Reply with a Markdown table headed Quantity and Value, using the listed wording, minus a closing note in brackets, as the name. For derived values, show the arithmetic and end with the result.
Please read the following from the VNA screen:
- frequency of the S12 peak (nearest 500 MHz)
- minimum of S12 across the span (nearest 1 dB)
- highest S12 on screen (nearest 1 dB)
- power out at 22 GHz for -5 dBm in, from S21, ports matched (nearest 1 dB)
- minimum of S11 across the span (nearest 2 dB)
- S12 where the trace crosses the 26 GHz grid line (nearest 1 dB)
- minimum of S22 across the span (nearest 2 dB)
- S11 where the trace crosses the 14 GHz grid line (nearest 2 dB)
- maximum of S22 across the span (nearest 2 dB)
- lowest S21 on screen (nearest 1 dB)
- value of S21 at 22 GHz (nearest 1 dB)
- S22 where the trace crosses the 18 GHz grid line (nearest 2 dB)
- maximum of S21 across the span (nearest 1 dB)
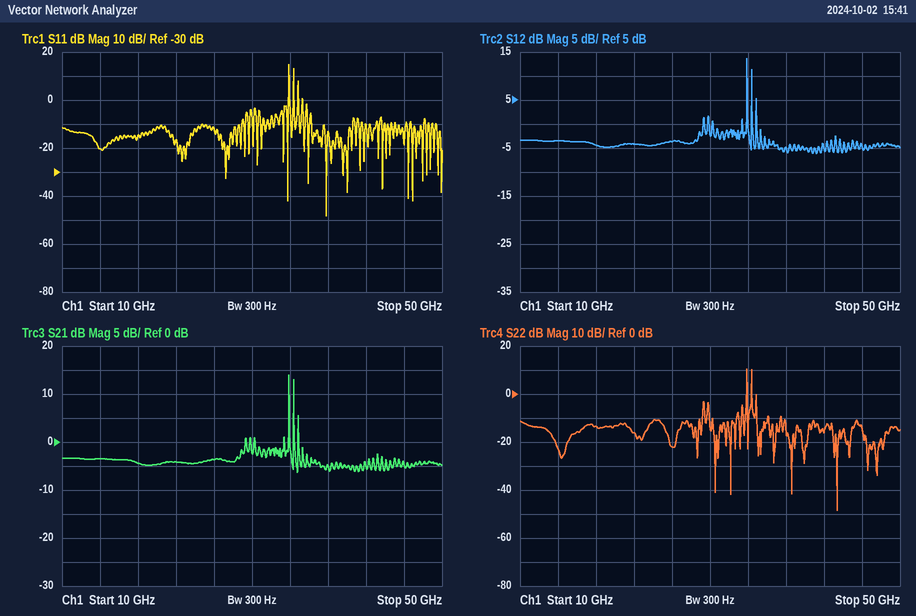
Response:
| Quantity | Value |
|---|---|
| frequency of the S12 peak | 34.0 GHz |
| minimum of S12 across the span | -6 dB |
| highest S12 on screen | 14 dB |
| power out at 22 GHz for -5 dBm in, from S21, ports matched | -5 dBm + (-4 dB) = -9 dBm |
| minimum of S11 across the span | -48 dB |
| S12 where the trace crosses the 26 GHz grid line | -4 dB |
| minimum of S22 across the span | -48 dB |
| S11 where the trace crosses the 14 GHz grid line | -20 dB |
| maximum of S22 across the span | 10 dB |
| lowest S21 on screen | -6 dB |
| value of S21 at 22 GHz | -4 dB |
| S22 where the trace crosses the 18 GHz grid line | -14 dB |
| maximum of S21 across the span | 14 dB |
